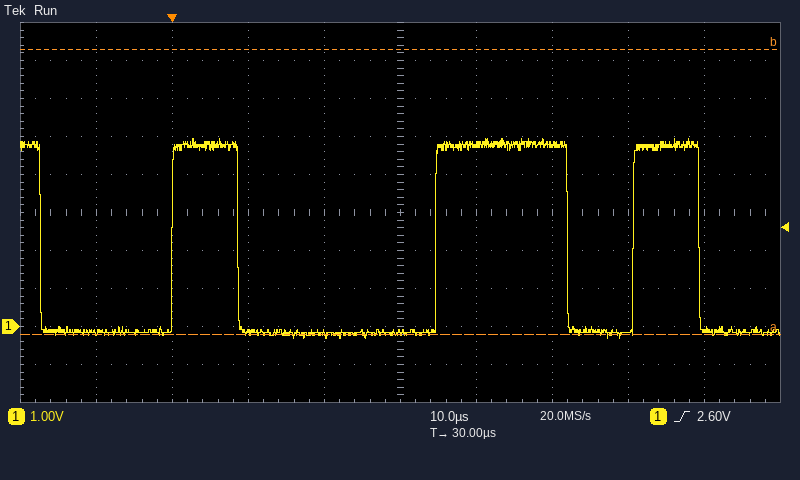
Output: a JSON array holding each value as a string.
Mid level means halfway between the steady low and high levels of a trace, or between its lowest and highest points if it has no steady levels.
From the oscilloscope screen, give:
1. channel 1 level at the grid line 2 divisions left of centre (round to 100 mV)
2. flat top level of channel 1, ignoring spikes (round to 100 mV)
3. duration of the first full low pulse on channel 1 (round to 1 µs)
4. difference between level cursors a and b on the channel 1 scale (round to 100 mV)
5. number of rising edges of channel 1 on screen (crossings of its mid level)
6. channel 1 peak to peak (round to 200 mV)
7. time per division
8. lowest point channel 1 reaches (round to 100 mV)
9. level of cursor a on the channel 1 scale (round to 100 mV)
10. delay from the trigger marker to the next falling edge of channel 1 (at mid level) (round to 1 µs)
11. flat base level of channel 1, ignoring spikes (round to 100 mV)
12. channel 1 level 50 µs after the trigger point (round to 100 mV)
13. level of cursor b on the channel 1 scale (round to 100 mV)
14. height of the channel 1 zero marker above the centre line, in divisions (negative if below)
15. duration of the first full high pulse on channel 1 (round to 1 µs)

["-200 mV", "4.8 V", "17 µs", "7.5 V", "3", "5.2 V", "10 µs", "-300 mV", "-200 mV", "9 µs", "-200 mV", "4.8 V", "7.3 V", "-3.0 div", "9 µs"]
